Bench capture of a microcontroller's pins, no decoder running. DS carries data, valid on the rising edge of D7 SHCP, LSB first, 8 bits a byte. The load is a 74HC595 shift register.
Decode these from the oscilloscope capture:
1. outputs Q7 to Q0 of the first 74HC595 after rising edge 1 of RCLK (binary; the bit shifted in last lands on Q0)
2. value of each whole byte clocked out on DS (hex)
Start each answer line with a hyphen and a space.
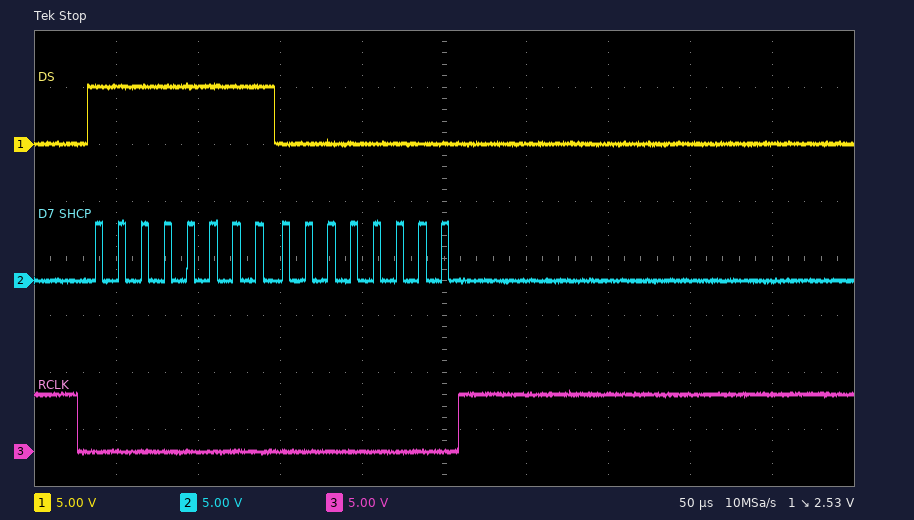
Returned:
- 00000000
- FF 00
